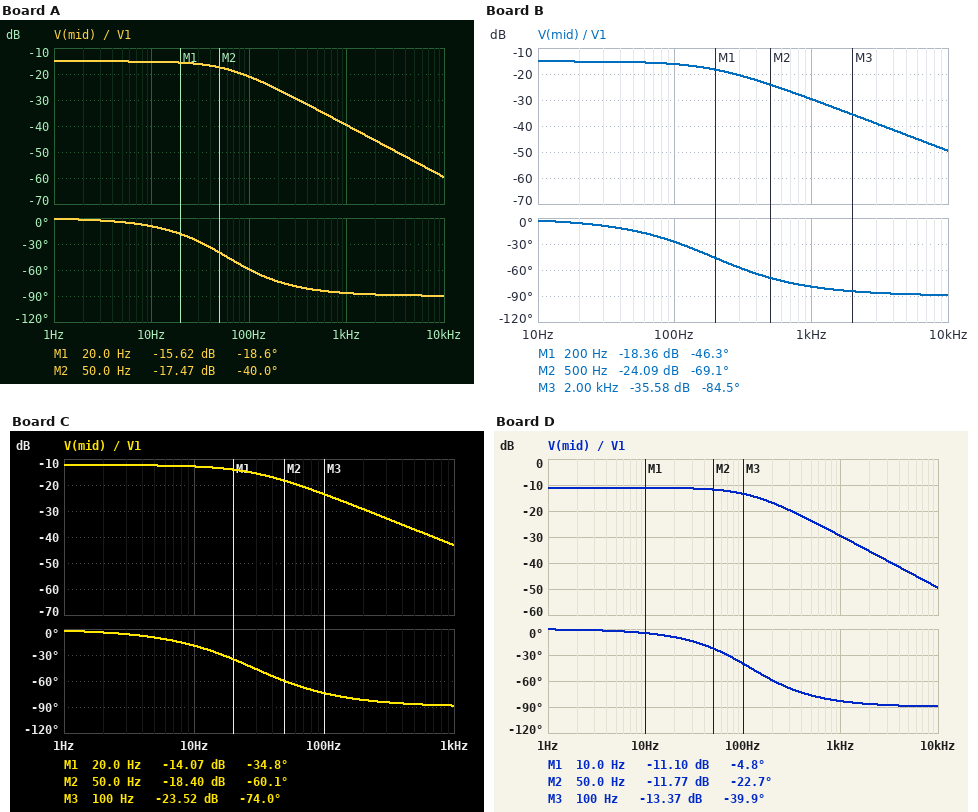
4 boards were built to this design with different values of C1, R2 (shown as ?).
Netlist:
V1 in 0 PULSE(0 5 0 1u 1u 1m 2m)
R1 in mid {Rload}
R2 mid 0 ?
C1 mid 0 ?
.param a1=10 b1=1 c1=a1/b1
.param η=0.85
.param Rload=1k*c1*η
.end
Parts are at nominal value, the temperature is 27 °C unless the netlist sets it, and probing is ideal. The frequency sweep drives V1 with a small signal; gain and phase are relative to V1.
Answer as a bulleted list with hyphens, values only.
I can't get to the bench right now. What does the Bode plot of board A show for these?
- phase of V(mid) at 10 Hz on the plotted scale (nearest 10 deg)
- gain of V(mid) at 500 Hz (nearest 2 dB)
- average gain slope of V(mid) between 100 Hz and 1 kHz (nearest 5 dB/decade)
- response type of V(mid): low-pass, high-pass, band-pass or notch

- -10 deg
- -34 dB
- -20 dB/decade
- low-pass
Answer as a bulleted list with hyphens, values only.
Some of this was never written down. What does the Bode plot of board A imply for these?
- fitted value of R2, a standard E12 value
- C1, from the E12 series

- 1.8 kΩ
- 1.8 µF
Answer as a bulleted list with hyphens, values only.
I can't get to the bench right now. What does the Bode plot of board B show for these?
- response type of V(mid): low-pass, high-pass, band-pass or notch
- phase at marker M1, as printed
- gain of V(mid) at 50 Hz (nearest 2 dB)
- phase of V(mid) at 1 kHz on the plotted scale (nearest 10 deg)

- low-pass
- -46.3 deg
- -16 dB
- -80 deg
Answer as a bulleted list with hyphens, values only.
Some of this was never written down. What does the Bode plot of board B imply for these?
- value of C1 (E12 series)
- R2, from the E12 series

- 560 nF
- 1.8 kΩ
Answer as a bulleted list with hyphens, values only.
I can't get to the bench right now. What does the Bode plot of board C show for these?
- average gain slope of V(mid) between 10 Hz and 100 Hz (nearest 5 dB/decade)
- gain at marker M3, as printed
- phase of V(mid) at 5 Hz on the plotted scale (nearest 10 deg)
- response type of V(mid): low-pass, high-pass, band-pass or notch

- -10 dB/decade
- -23.52 dB
- -10 deg
- low-pass
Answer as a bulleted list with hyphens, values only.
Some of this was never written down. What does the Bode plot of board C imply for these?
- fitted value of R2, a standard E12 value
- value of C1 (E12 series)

- 2.7 kΩ
- 2.7 µF
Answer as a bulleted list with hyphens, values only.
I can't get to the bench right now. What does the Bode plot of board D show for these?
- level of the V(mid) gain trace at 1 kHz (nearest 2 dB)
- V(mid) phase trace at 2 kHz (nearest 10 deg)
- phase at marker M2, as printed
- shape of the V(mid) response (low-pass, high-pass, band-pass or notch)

- -30 dB
- -90 deg
- -22.7 deg
- low-pass
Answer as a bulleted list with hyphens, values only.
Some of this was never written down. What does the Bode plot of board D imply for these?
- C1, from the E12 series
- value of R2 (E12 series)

- 560 nF
- 3.3 kΩ
